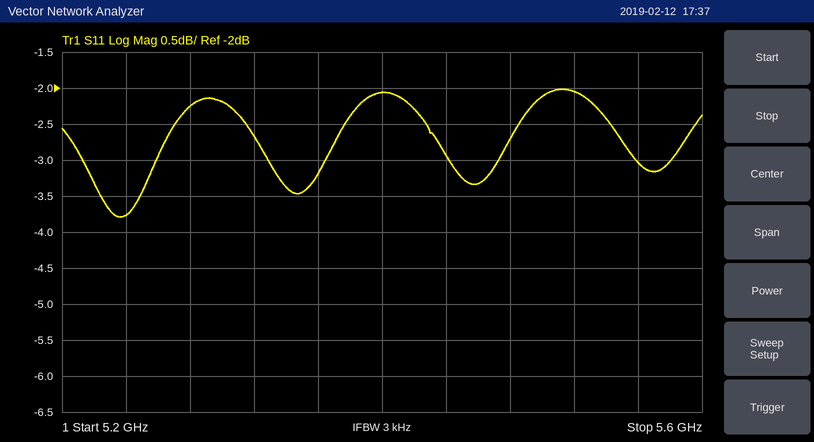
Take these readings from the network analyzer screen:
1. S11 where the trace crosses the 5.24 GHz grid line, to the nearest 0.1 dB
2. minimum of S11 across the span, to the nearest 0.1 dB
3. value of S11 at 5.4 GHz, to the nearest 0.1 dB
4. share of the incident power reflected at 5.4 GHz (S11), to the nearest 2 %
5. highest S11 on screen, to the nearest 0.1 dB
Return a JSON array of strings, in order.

["-3.8 dB", "-3.8 dB", "-2.1 dB", "62 %", "-2.0 dB"]
